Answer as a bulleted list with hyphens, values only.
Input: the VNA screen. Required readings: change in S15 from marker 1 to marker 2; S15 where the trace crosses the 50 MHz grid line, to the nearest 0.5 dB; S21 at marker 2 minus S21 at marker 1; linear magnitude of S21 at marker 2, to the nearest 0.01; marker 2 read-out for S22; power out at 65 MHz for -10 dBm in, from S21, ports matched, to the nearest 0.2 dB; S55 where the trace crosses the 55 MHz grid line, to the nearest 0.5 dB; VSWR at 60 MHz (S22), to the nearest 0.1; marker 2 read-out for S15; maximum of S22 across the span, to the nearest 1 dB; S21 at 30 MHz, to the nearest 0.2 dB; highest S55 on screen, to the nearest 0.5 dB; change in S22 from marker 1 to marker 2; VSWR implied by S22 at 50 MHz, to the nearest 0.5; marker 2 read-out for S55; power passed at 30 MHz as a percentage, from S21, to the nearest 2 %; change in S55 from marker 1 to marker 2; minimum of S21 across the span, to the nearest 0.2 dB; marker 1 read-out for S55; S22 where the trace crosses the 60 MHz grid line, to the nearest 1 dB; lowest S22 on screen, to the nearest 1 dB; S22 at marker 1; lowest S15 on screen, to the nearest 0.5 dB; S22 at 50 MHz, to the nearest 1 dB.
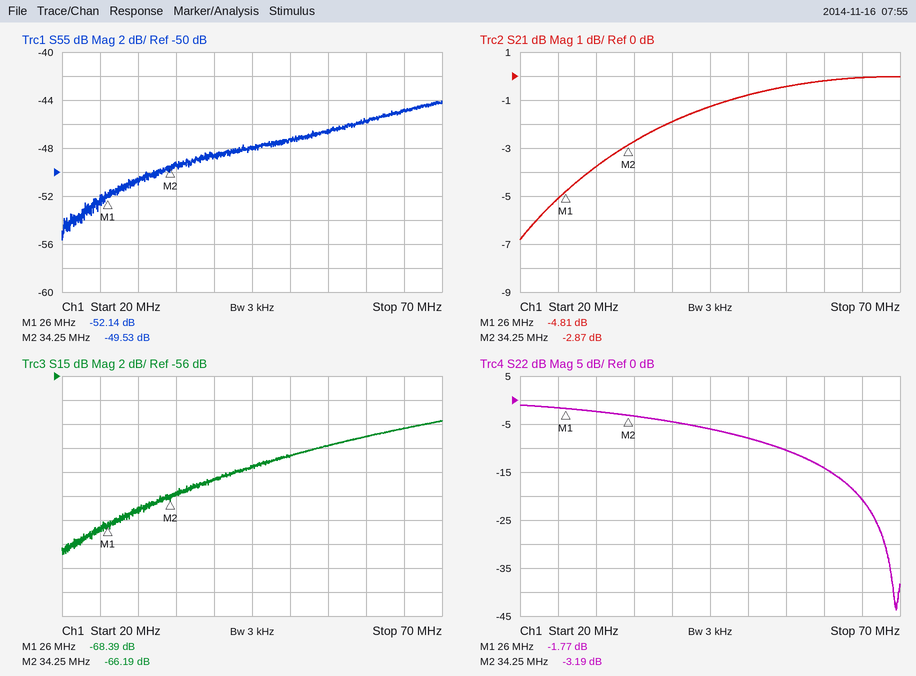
- 2.20 dB
- -62.5 dB
- 1.94 dB
- 0.72
- -3.19 dB
- -10.0 dBm
- -46.5 dB
- 1.5
- -66.19 dB
- -1 dB
- -3.8 dB
- -44.0 dB
- -1.42 dB
- 2.5
- -49.53 dB
- 42 %
- 2.61 dB
- -6.8 dB
- -52.14 dB
- -14 dB
- -44 dB
- -1.77 dB
- -71.0 dB
- -8 dB
